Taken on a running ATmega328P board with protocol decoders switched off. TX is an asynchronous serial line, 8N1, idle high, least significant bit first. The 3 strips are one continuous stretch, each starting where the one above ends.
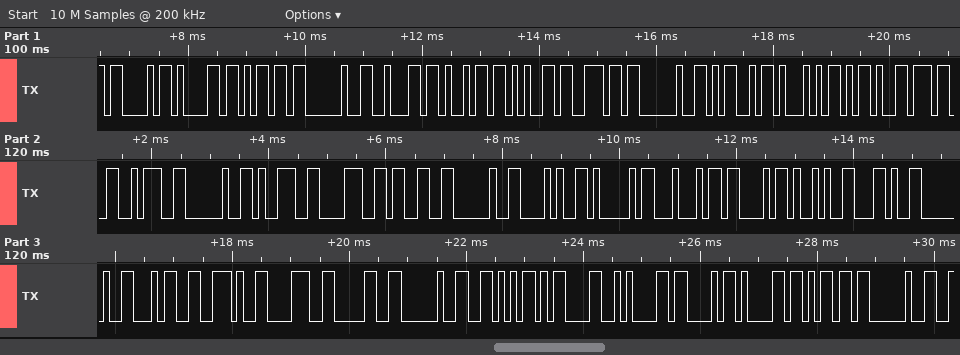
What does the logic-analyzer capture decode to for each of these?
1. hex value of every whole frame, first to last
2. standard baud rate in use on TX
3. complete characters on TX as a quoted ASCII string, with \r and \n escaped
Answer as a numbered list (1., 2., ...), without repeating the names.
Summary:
1. 43 61 6D 20 62 69 65 6E 20 4D 51 2D 37 3A 20 39 38 33 20 28 41 44 43 29 2C 20 34 2E 38 30 20 56 0D 0A 43 61 6D 20
2. 9600 baud
3. "Cam bien MQ-7: 983 (ADC), 4.80 V\r\nCam "
